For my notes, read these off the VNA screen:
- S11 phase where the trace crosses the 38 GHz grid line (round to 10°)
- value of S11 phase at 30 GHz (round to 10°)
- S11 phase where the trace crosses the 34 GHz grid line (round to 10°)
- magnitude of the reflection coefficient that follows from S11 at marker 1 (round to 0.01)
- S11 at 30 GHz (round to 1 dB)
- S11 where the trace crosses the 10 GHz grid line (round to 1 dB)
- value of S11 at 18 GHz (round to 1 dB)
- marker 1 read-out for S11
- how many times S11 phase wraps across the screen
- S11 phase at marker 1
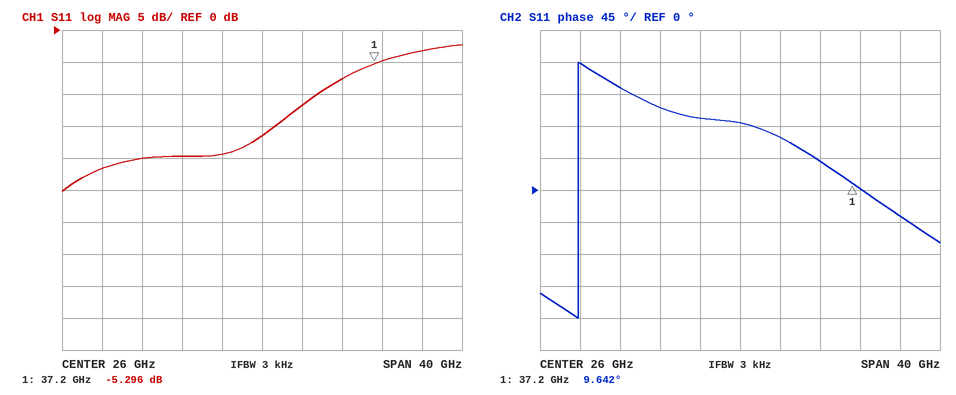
0°
70°
40°
0.54
-12 dB
-22 dB
-20 dB
-5.296 dB
1
9.642°
